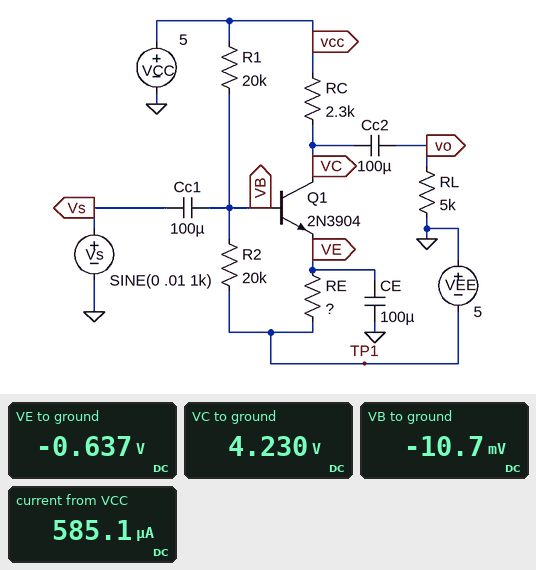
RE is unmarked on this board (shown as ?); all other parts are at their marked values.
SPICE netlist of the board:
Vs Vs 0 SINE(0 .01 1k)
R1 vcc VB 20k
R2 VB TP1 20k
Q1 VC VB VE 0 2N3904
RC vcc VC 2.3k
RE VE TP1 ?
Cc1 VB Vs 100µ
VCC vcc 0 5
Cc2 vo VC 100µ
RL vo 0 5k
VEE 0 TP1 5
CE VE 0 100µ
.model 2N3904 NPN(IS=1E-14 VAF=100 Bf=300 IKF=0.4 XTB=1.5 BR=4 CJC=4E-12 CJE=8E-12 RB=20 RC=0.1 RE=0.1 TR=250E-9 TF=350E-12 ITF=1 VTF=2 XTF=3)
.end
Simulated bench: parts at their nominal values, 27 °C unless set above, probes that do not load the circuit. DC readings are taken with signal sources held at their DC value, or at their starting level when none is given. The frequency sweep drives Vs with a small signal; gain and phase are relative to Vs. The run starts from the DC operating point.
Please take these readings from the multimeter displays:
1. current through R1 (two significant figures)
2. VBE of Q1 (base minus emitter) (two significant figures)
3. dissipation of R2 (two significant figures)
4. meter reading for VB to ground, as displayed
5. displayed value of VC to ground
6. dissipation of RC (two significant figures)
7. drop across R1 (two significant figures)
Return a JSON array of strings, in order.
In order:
["250 µA", "630 mV", "1.2 mW", "-10.7 mV", "4.230 V", "260 µW", "5.0 V"]
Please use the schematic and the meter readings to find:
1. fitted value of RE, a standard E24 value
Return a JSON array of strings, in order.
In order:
["13 kΩ"]
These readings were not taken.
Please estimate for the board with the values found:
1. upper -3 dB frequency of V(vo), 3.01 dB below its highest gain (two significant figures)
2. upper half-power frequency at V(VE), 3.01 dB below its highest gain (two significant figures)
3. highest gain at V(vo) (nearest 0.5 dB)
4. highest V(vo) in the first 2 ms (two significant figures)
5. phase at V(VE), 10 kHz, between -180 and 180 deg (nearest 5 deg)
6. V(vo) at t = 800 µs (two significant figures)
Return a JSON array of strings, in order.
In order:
["37 MHz", "21 Hz", "26.0 dB", "170 mV", "-90 deg", "160 mV"]
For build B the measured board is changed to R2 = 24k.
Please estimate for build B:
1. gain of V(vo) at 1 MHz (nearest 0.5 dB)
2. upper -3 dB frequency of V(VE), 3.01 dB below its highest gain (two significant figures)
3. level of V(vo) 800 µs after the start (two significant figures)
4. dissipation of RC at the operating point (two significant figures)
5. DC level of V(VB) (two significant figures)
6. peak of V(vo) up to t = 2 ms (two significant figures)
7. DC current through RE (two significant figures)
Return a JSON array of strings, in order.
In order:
["27.0 dB", "23 Hz", "180 mV", "310 µW", "440 mV", "190 mV", "370 µA"]
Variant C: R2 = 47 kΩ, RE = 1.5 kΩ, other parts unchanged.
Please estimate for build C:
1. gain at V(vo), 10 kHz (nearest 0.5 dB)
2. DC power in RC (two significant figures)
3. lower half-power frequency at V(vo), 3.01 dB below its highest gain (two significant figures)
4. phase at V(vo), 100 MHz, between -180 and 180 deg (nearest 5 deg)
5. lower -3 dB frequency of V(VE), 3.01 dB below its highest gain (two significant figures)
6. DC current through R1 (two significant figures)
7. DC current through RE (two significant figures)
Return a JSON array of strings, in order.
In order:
["7.0 dB", "15 mW", "55 Hz", "-10 deg", "1.0 Hz", "260 µA", "2.7 mA"]
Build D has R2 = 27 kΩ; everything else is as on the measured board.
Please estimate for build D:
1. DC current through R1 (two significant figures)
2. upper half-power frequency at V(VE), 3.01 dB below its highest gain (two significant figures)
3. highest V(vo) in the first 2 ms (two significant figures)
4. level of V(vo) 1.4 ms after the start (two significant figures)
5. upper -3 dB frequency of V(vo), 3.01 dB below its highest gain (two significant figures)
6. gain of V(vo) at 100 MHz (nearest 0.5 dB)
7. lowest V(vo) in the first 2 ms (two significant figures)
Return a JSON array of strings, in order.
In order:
["210 µA", "24 Hz", "200 mV", "-140 mV", "33 MHz", "17.5 dB", "-280 mV"]
